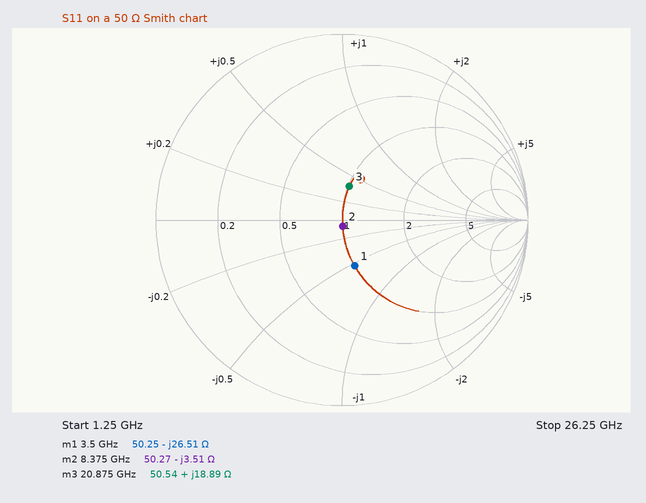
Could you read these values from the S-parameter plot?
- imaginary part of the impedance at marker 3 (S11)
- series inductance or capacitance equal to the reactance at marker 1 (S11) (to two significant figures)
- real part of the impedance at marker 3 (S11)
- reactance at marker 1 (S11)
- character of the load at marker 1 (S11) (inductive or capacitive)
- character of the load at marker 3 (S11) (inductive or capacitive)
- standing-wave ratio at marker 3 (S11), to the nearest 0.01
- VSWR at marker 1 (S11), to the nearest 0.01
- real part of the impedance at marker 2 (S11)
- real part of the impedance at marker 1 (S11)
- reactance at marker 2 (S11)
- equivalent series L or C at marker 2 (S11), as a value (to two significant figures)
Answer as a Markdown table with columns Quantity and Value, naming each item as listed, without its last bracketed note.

| Quantity | Value |
|---|---|
| imaginary part of the impedance at marker 3 | +18.89 Ω |
| series inductance or capacitance equal to the reactance at marker 1 (S11) | 1.7 pF |
| real part of the impedance at marker 3 | 50.54 Ω |
| reactance at marker 1 | -26.51 Ω |
| character of the load at marker 1 (S11) | capacitive |
| character of the load at marker 3 (S11) | inductive |
| standing-wave ratio at marker 3 (S11), to the nearest 0.01 | 1.45 |
| VSWR at marker 1 (S11), to the nearest 0.01 | 1.69 |
| real part of the impedance at marker 2 | 50.27 Ω |
| real part of the impedance at marker 1 | 50.25 Ω |
| reactance at marker 2 | -3.51 Ω |
| equivalent series L or C at marker 2 (S11), as a value | 5.4 pF |
